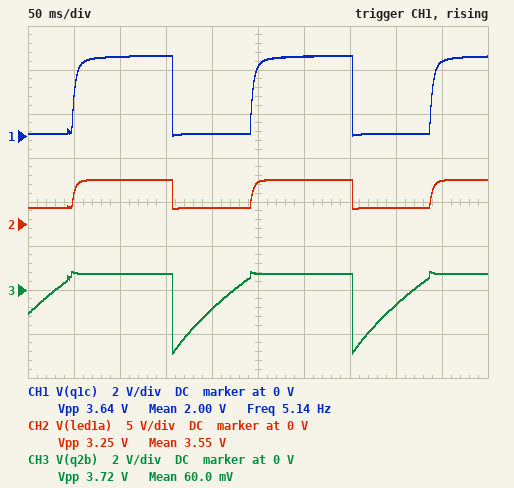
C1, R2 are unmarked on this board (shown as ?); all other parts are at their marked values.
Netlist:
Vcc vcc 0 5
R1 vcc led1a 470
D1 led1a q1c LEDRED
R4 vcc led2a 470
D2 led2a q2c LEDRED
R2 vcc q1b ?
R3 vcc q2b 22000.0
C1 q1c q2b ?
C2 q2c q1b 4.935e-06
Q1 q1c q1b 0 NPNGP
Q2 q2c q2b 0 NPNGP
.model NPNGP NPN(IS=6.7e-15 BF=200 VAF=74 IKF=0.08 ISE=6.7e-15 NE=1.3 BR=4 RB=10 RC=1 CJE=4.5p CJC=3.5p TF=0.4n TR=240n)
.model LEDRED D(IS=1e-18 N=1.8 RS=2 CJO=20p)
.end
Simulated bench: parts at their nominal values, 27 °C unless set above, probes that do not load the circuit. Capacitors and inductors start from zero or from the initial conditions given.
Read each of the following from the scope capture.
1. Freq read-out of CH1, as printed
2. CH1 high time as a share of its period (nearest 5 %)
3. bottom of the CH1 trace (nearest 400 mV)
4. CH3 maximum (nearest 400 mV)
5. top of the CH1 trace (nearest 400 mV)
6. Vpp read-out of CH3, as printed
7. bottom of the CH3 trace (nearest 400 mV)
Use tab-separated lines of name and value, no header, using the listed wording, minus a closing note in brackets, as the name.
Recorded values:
Freq read-out of CH1, as printed	5.14 Hz
CH1 high time as a share of its period	55 %
bottom of the CH1 trace	0 V
CH3 maximum	800 mV
top of the CH1 trace	3.6 V
Vpp read-out of CH3, as printed	3.72 V
bottom of the CH3 trace	-2.8 V
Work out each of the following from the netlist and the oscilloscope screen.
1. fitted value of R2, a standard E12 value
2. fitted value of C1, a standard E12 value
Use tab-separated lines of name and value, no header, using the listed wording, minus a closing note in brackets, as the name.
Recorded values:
fitted value of R2, a standard E12 value	39 kΩ
fitted value of C1, a standard E12 value	6.8 µF
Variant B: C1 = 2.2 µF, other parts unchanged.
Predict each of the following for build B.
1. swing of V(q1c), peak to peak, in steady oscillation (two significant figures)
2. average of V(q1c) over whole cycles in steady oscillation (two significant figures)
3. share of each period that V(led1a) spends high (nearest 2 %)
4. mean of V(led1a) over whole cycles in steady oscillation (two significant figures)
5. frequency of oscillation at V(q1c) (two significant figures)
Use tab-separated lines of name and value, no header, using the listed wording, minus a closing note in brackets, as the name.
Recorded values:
swing of V(q1c), peak to peak, in steady oscillation	3.7 V
average of V(q1c) over whole cycles in steady oscillation	2.9 V
share of each period that V(led1a) spends high	80 %
mean of V(led1a) over whole cycles in steady oscillation	4.3 V
frequency of oscillation at V(q1c)	7.3 Hz
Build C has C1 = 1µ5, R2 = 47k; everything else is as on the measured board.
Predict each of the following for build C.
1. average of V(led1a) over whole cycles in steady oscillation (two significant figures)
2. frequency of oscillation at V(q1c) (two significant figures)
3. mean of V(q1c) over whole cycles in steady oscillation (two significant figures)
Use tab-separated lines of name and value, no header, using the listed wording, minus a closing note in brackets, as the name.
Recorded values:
average of V(led1a) over whole cycles in steady oscillation	4.6 V
frequency of oscillation at V(q1c)	6.7 Hz
mean of V(q1c) over whole cycles in steady oscillation	3.2 V
